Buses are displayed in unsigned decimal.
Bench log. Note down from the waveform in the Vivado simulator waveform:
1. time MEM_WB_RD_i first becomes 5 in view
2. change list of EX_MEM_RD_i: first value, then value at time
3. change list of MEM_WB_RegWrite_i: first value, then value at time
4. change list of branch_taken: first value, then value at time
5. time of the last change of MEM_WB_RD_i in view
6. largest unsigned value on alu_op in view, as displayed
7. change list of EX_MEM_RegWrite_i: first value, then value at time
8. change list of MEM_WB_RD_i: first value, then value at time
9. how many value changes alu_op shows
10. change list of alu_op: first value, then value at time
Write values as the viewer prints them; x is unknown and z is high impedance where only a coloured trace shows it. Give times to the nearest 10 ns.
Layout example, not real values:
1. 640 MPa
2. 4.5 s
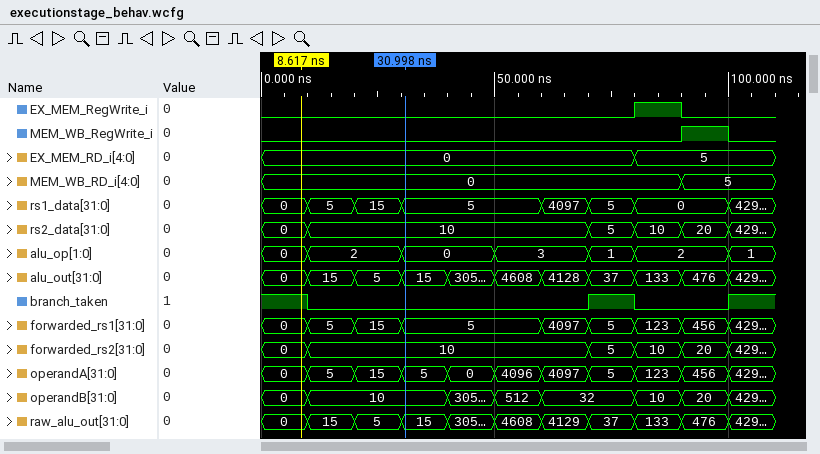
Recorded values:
1. 90 ns
2. 0, 5 at 80 ns
3. 0, 1 at 90 ns, 0 at 100 ns
4. 1, 0 at 10 ns, 1 at 70 ns, 0 at 80 ns, 1 at 100 ns
5. 90 ns
6. 3
7. 0, 1 at 80 ns, 0 at 90 ns
8. 0, 5 at 90 ns
9. 6
10. 0, 2 at 10 ns, 0 at 30 ns, 3 at 50 ns, 1 at 70 ns, 2 at 80 ns, 1 at 100 ns
